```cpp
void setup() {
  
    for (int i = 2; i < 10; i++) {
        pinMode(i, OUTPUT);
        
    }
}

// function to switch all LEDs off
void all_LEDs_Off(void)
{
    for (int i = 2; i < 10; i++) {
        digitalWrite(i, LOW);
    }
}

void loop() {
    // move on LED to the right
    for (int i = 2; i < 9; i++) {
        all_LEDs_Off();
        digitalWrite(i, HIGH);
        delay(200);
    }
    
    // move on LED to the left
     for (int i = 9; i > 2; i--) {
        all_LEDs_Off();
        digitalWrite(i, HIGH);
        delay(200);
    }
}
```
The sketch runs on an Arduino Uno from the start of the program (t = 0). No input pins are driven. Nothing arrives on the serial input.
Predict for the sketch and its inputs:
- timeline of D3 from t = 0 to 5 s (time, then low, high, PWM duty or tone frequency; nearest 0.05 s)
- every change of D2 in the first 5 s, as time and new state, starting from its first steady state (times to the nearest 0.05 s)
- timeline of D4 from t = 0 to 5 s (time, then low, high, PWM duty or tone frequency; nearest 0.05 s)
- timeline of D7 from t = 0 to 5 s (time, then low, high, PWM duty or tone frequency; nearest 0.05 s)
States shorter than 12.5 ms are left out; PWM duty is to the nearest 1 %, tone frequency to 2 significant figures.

0 s low; 0.2 s high; 0.4 s low; 2.6 s high; 2.8 s low; 3 s high; 3.2 s low
0 s high; 0.2 s low; 2.8 s high; 3 s low
0 s low; 0.4 s high; 0.6 s low; 2.4 s high; 2.6 s low; 3.2 s high; 3.4 s low
0 s low; 1 s high; 1.2 s low; 1.8 s high; 2 s low; 3.8 s high; 4 s low; 4.6 s high; 4.8 s low
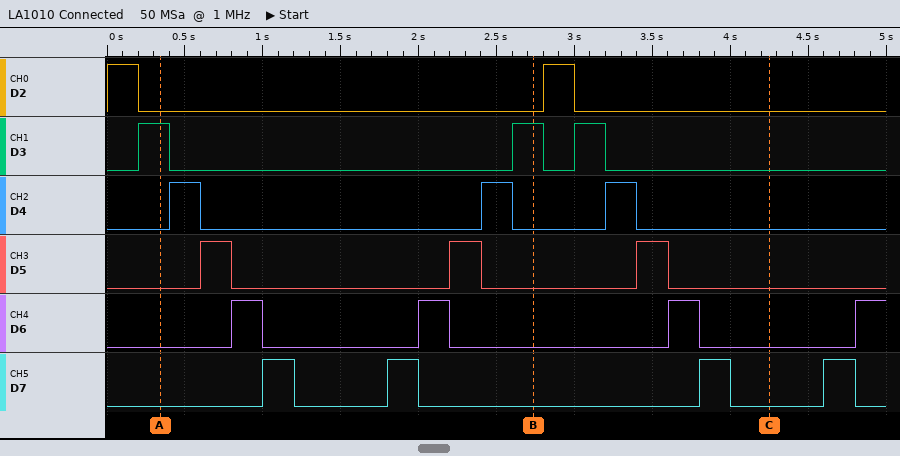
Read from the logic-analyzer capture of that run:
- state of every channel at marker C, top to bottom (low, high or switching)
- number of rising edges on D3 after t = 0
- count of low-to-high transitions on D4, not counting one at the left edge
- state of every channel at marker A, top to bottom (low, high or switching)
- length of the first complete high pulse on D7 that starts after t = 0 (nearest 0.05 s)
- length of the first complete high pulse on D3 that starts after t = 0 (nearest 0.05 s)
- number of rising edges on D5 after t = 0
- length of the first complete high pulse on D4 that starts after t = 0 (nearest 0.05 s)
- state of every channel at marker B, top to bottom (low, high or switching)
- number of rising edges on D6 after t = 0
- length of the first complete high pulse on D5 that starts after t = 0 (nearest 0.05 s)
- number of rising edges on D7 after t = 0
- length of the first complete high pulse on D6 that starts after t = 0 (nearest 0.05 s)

D2 low, D3 low, D4 low, D5 low, D6 low, D7 low
3
3
D2 low, D3 high, D4 low, D5 low, D6 low, D7 low
0.20 s
0.20 s
3
0.20 s
D2 low, D3 high, D4 low, D5 low, D6 low, D7 low
4
0.20 s
4
0.20 s
